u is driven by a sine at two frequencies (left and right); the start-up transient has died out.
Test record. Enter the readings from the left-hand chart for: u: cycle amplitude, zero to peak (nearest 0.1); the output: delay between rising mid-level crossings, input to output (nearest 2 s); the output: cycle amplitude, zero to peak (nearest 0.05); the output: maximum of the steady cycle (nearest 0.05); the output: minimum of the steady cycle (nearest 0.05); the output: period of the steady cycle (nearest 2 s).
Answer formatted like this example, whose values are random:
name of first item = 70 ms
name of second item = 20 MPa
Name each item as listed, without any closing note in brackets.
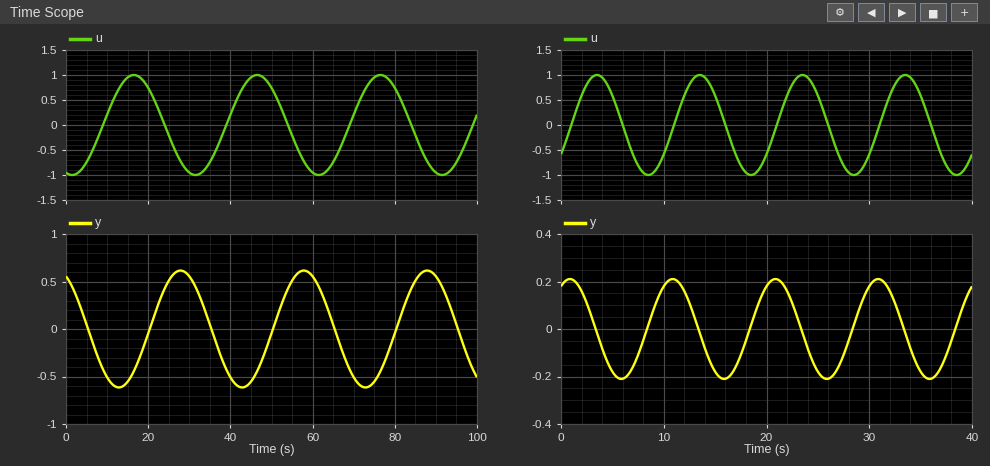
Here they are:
u: cycle amplitude, zero to peak = 1.0
the output: delay between rising mid-level crossings, input to output = 12 s
the output: cycle amplitude, zero to peak = 0.60
the output: maximum of the steady cycle = 0.60
the output: minimum of the steady cycle = -0.60
the output: period of the steady cycle = 30 s
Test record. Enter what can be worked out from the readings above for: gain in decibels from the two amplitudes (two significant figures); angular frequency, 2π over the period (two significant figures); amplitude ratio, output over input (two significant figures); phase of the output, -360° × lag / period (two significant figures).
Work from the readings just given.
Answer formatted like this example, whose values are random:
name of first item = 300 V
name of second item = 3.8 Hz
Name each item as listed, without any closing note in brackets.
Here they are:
gain in decibels from the two amplitudes = -4.4 dB
angular frequency, 2π over the period = 0.21 rad/s
amplitude ratio, output over input = 0.60
phase of the output, -360° × lag / period = -140°
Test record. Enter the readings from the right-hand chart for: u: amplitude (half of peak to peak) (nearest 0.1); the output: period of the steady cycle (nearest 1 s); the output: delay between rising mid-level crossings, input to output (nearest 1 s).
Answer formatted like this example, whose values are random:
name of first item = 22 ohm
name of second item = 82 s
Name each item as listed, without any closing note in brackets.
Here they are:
u: amplitude (half of peak to peak) = 1.0
the output: period of the steady cycle = 10 s
the output: delay between rising mid-level crossings, input to output = 7 s
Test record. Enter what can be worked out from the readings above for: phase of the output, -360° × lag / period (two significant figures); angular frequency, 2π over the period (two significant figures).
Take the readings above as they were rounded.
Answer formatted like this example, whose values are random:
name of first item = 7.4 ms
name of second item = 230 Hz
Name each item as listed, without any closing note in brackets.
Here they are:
phase of the output, -360° × lag / period = -250°
angular frequency, 2π over the period = 0.63 rad/s
